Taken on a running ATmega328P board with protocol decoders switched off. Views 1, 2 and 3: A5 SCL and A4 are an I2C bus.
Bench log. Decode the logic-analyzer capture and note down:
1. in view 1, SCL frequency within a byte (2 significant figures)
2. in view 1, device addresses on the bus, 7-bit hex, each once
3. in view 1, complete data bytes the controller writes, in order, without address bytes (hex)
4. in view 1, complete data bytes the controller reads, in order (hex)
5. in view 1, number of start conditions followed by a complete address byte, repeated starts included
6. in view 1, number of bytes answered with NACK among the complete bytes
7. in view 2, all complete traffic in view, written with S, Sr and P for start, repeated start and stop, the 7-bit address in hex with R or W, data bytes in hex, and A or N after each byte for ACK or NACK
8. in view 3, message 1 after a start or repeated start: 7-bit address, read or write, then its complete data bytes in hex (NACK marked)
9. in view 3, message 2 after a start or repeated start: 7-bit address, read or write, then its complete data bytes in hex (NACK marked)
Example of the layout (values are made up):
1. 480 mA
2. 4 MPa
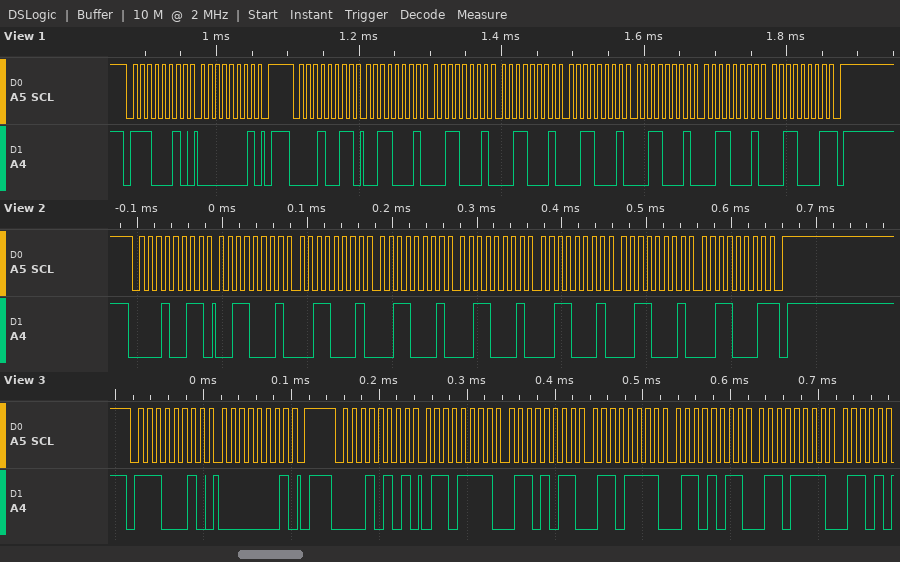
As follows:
1. 100 kHz
2. 0x71 0x09
3. 01
4. 31 31 31 31 31 31 31
5. 2
6. 1
7. S 09R A 31 A 31 A 31 A 31 A 31 A 31 A 31 N P
8. 0x71 write: 01
9. 0x0A read: 6F 6B 6F 6B 6F
